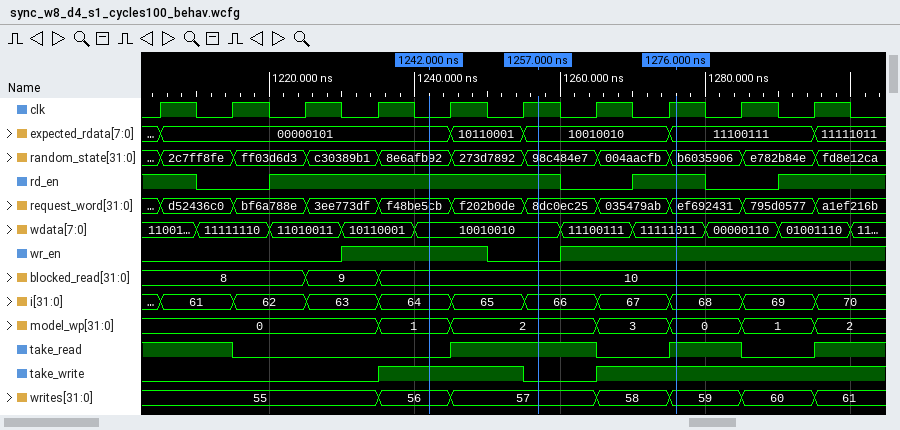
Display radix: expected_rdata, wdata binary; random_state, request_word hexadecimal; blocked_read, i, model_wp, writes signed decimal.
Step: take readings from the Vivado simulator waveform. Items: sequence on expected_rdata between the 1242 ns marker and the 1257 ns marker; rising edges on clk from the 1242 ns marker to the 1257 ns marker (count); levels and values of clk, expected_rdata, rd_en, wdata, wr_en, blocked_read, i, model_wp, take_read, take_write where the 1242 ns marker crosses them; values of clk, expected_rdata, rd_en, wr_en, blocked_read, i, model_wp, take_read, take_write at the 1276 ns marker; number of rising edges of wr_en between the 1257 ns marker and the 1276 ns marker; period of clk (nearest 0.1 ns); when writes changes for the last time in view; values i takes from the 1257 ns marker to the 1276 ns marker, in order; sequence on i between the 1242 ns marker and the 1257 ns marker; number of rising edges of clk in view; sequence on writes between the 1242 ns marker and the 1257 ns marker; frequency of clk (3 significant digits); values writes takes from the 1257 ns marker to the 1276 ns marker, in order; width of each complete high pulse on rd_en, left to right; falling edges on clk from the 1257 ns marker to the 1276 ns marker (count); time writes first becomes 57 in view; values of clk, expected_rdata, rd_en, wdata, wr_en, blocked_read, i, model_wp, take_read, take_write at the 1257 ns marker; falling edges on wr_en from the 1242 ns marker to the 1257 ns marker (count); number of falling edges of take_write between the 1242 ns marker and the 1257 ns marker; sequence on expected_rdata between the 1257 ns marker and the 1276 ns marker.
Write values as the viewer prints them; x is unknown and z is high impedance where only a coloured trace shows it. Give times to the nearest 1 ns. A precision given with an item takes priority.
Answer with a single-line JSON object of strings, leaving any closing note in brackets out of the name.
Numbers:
{"sequence on expected_rdata between the 1242 ns marker and the 1257 ns marker": "00000101, 10110001, 10010010", "rising edges on clk from the 1242 ns marker to the 1257 ns marker": "2", "levels and values of clk, expected_rdata, rd_en, wdata, wr_en, blocked_read, i, model_wp, take_read, take_write where the 1242 ns marker crosses them": "clk=0, expected_rdata=00000101, rd_en=1, wdata=10010010, wr_en=1, blocked_read=10, i=64, model_wp=1, take_read=0, take_write=1", "values of clk, expected_rdata, rd_en, wr_en, blocked_read, i, model_wp, take_read, take_write at the 1276 ns marker": "clk=1, expected_rdata=11100111, rd_en=1, wr_en=1, blocked_read=10, i=68, model_wp=0, take_read=1, take_write=1", "number of rising edges of wr_en between the 1257 ns marker and the 1276 ns marker": "1", "period of clk": "10 ns", "when writes changes for the last time in view": "1295 ns", "values i takes from the 1257 ns marker to the 1276 ns marker, in order": "66, 67, 68", "sequence on i between the 1242 ns marker and the 1257 ns marker": "64, 65, 66", "number of rising edges of clk in view": "10", "sequence on writes between the 1242 ns marker and the 1257 ns marker": "56, 57", "frequency of clk": "100 MHz", "values writes takes from the 1257 ns marker to the 1276 ns marker, in order": "57, 58, 59", "width of each complete high pulse on rd_en, left to right": "40 ns, 10 ns", "falling edges on clk from the 1257 ns marker to the 1276 ns marker": "2", "time writes first becomes 57 in view": "1245 ns", "values of clk, expected_rdata, rd_en, wdata, wr_en, blocked_read, i, model_wp, take_read, take_write at the 1257 ns marker": "clk=1, expected_rdata=10010010, rd_en=1, wdata=10010010, wr_en=0, blocked_read=10, i=66, model_wp=2, take_read=1, take_write=0", "falling edges on wr_en from the 1242 ns marker to the 1257 ns marker": "1", "number of falling edges of take_write between the 1242 ns marker and the 1257 ns marker": "1", "sequence on expected_rdata between the 1257 ns marker and the 1276 ns marker": "10010010, 11100111"}
